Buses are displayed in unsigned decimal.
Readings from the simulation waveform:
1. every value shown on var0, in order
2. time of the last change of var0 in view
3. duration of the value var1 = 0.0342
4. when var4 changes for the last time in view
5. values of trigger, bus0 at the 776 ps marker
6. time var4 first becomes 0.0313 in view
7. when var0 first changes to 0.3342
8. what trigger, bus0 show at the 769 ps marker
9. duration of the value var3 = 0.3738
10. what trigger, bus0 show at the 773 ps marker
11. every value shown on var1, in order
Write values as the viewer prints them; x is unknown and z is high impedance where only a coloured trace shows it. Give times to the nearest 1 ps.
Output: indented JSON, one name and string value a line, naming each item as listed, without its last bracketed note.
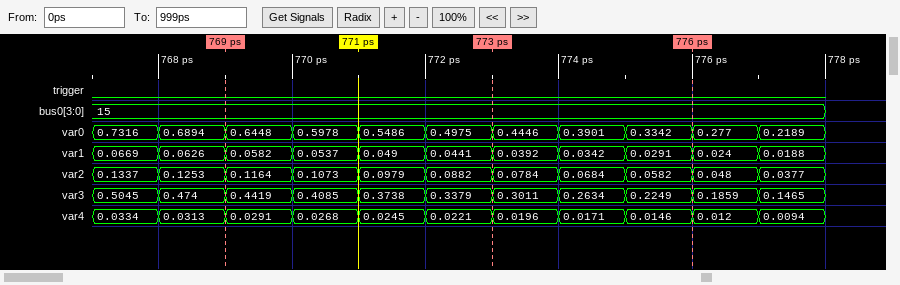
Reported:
{
  "every value shown on var0, in order": "0.7316, 0.6894, 0.6448, 0.5978, 0.5486, 0.4975, 0.4446, 0.3901, 0.3342, 0.277, 0.2189",
  "time of the last change of var0 in view": "777 ps",
  "duration of the value var1 = 0.0342": "1 ps",
  "when var4 changes for the last time in view": "777 ps",
  "values of trigger, bus0 at the 776 ps marker": "trigger=0, bus0=15",
  "time var4 first becomes 0.0313 in view": "768 ps",
  "when var0 first changes to 0.3342": "775 ps",
  "what trigger, bus0 show at the 769 ps marker": "trigger=0, bus0=15",
  "duration of the value var3 = 0.3738": "1 ps",
  "what trigger, bus0 show at the 773 ps marker": "trigger=0, bus0=15",
  "every value shown on var1, in order": "0.0669, 0.0626, 0.0582, 0.0537, 0.049, 0.0441, 0.0392, 0.0342, 0.0291, 0.024, 0.0188"
}
